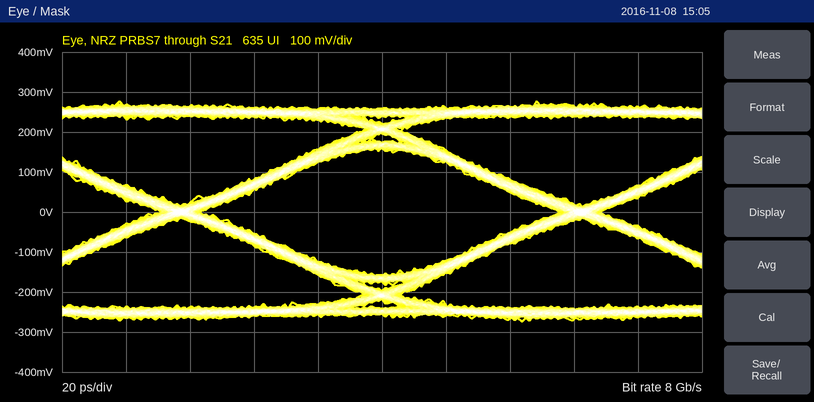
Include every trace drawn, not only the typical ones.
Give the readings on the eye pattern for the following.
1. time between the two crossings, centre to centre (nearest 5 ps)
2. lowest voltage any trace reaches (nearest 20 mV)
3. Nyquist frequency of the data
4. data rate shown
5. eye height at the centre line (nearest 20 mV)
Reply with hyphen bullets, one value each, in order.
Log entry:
- 125 ps
- -280 mV
- 4 GHz
- 8 Gb/s
- 320 mV
